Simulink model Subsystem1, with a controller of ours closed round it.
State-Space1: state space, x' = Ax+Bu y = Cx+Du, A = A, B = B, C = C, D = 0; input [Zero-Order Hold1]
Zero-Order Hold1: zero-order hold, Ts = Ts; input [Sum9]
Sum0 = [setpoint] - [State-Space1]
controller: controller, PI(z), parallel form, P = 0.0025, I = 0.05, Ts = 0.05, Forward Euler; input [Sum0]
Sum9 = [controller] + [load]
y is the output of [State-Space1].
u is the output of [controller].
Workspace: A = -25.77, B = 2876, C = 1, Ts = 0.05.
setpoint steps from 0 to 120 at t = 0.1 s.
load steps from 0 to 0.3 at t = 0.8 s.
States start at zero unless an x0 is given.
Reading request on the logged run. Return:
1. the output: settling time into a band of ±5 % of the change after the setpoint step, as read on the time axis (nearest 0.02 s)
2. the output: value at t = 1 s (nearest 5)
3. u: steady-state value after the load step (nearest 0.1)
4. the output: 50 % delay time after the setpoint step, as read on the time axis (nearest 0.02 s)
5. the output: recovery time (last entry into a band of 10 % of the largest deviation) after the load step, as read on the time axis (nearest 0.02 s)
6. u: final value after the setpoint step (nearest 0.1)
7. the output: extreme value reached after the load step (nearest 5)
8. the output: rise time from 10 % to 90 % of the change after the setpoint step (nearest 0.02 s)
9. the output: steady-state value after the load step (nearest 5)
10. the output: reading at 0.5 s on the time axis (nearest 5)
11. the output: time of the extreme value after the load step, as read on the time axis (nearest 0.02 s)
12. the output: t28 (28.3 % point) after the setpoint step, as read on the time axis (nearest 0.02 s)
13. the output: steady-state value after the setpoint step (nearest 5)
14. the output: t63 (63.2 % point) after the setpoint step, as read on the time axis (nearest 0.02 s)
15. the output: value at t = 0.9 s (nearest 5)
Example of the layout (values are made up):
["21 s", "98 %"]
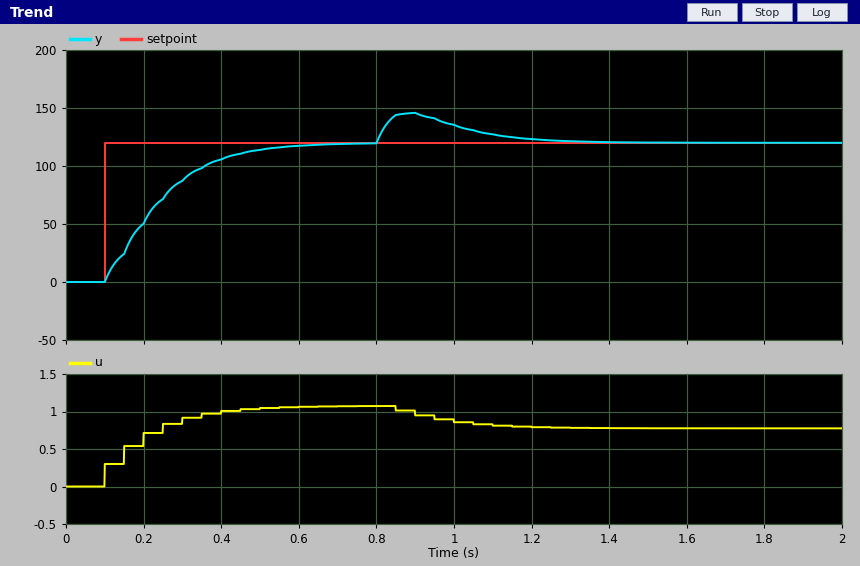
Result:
["0.50 s", "135", "0.8", "0.22 s", "1.22 s", "1.1", "145", "0.30 s", "120", "115", "0.90 s", "0.16 s", "120", "0.26 s", "145"]
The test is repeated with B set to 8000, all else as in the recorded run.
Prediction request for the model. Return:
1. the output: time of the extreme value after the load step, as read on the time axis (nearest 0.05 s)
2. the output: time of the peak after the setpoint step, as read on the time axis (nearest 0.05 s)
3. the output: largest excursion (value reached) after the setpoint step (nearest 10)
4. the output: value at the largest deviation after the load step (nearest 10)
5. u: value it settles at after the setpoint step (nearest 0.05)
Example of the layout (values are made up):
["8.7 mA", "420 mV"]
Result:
["0.85 s", "0.25 s", "130", "190", "0.40"]
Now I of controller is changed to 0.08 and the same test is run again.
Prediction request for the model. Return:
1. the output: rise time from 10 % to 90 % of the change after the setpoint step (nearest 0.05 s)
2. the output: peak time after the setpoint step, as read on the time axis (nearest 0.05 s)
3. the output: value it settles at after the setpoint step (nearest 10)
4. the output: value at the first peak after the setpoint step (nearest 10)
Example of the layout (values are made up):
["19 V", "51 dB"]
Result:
["0.15 s", "0.40 s", "120", "130"]
